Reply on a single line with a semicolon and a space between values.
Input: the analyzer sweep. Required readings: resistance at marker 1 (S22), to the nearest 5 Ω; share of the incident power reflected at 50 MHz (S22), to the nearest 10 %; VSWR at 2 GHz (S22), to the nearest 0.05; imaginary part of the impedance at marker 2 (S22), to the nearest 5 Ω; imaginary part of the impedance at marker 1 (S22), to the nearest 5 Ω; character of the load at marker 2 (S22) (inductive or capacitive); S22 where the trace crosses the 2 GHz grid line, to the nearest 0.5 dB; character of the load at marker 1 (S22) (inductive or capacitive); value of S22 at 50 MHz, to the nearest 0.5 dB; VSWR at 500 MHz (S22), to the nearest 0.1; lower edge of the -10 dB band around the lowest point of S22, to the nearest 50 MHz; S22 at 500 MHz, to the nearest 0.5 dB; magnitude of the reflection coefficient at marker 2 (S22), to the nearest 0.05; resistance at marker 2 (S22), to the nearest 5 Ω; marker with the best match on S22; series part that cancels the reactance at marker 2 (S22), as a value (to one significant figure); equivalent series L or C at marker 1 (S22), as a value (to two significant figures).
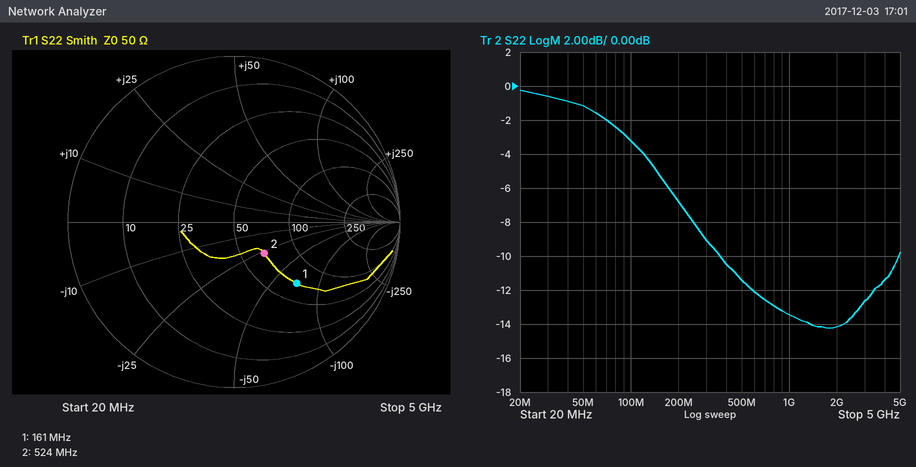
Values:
70 Ω; 80 %; 1.50; -25 Ω; -70 Ω; capacitive; -14.0 dB; capacitive; -1.0 dB; 1.7; 350 MHz; -11.5 dB; 0.25; 65 Ω; marker 2; 8 nH; 14 pF
